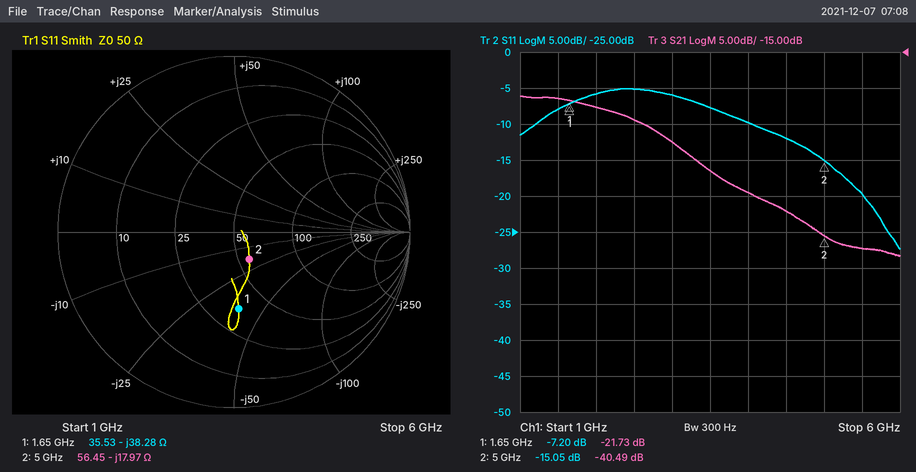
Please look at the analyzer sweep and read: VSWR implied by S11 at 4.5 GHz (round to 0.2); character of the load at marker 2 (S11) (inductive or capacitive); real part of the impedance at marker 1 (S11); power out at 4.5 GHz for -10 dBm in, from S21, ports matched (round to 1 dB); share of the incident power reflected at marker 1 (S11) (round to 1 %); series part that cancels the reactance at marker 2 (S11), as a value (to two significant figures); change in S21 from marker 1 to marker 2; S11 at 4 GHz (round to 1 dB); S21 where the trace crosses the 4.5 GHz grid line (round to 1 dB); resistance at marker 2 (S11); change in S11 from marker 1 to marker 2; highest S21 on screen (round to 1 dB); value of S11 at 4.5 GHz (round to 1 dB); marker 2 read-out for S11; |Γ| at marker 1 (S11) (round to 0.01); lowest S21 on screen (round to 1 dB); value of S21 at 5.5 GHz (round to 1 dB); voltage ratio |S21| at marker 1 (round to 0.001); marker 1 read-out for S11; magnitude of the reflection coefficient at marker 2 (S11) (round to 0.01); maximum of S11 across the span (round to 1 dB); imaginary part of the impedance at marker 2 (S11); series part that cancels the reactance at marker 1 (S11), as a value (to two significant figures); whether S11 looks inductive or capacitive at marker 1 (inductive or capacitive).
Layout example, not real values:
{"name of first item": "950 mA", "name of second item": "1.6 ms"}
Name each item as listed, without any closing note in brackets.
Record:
{"VSWR implied by S11 at 4.5 GHz": "1.6", "character of the load at marker 2 (S11)": "capacitive", "real part of the impedance at marker 1": "35.53 Ω", "power out at 4.5 GHz for -10 dBm in, from S21, ports matched": "-47 dBm", "share of the incident power reflected at marker 1 (S11)": "19 %", "series part that cancels the reactance at marker 2 (S11), as a value": "570 pH", "change in S21 from marker 1 to marker 2": "-18.76 dB", "S11 at 4 GHz": "-10 dB", "S21 where the trace crosses the 4.5 GHz grid line": "-37 dB", "resistance at marker 2": "56.45 Ω", "change in S11 from marker 1 to marker 2": "-7.85 dB", "highest S21 on screen": "-21 dB", "value of S11 at 4.5 GHz": "-12 dB", "marker 2 read-out for S11": "-15.05 dB", "|Γ| at marker 1 (S11)": "0.44", "lowest S21 on screen": "-43 dB", "value of S21 at 5.5 GHz": "-42 dB", "voltage ratio |S21| at marker 1": "0.082", "marker 1 read-out for S11": "-7.20 dB", "magnitude of the reflection coefficient at marker 2 (S11)": "0.18", "maximum of S11 across the span": "-5 dB", "imaginary part of the impedance at marker 2": "-17.97 Ω", "series part that cancels the reactance at marker 1 (S11), as a value": "3.7 nH", "whether S11 looks inductive or capacitive at marker 1": "capacitive"}
